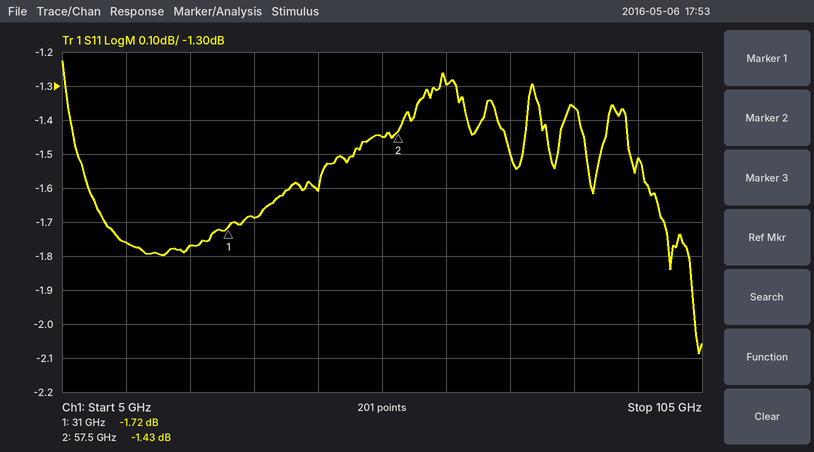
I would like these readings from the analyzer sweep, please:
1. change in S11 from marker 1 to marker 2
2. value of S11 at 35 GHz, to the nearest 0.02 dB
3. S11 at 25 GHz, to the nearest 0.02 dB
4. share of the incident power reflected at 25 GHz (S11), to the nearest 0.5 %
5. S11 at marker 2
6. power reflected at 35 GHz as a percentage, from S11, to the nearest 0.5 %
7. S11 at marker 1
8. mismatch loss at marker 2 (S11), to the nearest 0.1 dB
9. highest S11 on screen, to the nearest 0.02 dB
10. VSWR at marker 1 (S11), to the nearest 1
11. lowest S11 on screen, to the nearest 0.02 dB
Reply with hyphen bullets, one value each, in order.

- 0.29 dB
- -1.68 dB
- -1.76 dB
- 66.5 %
- -1.43 dB
- 68.0 %
- -1.72 dB
- 5.5 dB
- -1.22 dB
- 10
- -2.08 dB
